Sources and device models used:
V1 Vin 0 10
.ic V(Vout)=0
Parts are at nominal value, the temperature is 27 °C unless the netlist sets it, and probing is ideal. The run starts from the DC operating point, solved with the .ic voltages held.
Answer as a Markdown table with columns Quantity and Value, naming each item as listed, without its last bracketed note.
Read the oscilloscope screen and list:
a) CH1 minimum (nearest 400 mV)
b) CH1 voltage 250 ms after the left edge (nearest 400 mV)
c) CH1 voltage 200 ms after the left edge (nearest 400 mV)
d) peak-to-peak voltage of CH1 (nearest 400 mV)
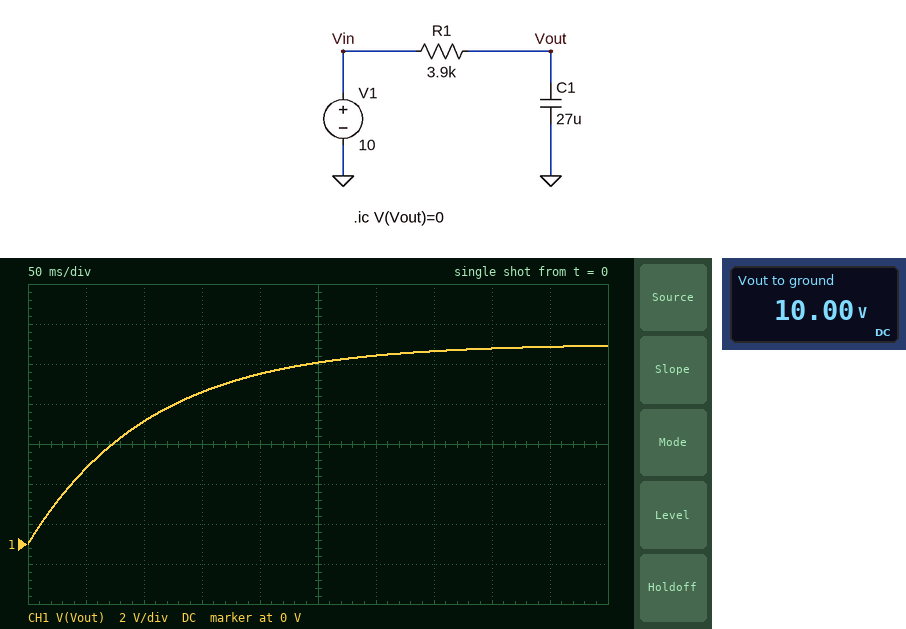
| Quantity | Value |
|---|---|
| CH1 minimum | 0 V |
| CH1 voltage 250 ms after the left edge | 9.2 V |
| CH1 voltage 200 ms after the left edge | 8.4 V |
| peak-to-peak voltage of CH1 | 10.0 V |
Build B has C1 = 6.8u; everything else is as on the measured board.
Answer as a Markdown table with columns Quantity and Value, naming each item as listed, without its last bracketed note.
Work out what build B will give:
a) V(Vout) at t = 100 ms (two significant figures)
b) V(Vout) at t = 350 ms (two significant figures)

| Quantity | Value |
|---|---|
| V(Vout) at t = 100 ms | 9.8 V |
| V(Vout) at t = 350 ms | 10 V |
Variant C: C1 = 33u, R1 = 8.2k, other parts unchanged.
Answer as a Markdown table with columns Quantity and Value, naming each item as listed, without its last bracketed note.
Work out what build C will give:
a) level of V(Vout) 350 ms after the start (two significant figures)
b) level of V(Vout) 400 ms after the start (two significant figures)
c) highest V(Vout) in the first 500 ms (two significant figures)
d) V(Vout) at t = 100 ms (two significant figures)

| Quantity | Value |
|---|---|
| level of V(Vout) 350 ms after the start | 7.3 V |
| level of V(Vout) 400 ms after the start | 7.7 V |
| highest V(Vout) in the first 500 ms | 8.4 V |
| V(Vout) at t = 100 ms | 3.1 V |
